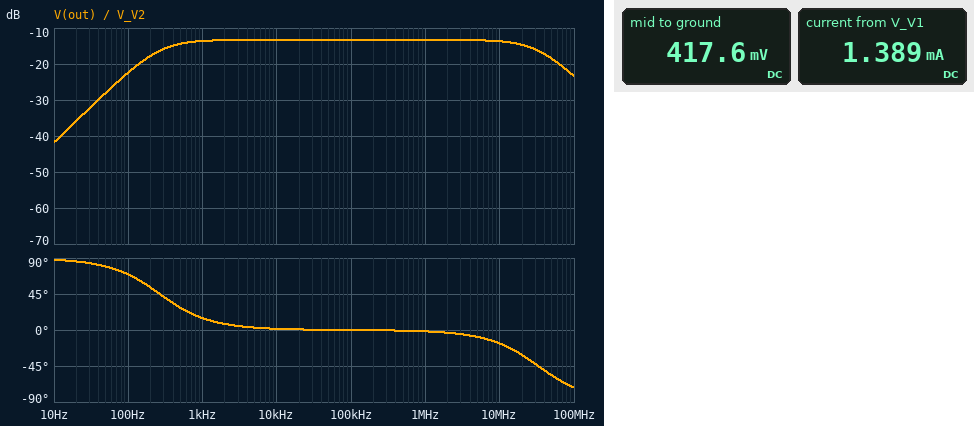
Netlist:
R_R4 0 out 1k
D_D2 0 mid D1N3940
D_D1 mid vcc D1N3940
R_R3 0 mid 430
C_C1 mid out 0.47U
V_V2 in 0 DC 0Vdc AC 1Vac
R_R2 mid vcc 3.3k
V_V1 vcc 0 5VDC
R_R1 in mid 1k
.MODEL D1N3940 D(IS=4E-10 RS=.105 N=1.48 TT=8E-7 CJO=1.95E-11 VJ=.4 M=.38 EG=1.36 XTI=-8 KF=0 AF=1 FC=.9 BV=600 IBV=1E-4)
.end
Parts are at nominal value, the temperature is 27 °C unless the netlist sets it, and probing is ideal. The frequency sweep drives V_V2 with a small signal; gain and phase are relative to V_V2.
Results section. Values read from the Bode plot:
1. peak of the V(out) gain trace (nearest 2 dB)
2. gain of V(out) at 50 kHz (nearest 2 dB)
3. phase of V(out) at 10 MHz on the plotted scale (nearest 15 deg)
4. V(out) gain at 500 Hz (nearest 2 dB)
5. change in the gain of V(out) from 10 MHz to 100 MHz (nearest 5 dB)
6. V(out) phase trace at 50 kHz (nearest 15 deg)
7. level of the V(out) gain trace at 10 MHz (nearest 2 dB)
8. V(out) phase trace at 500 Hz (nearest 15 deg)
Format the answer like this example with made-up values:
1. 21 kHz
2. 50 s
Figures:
1. -14 dB
2. -14 dB
3. -15 deg
4. -14 dB
5. -10 dB
6. 0 deg
7. -14 dB
8. 30 deg
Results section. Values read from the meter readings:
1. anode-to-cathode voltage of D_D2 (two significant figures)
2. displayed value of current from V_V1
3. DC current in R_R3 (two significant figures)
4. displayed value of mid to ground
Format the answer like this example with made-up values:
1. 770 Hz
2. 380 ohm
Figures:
1. -420 mV
2. 1.389 mA
3. 970 µA
4. 417.6 mV
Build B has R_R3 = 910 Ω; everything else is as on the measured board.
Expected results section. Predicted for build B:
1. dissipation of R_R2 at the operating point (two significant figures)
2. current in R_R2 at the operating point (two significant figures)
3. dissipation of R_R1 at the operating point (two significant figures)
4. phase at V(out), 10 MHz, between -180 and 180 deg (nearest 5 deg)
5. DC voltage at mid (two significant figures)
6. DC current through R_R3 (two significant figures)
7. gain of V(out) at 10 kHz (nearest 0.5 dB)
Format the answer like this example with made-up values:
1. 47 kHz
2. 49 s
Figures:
1. 5.8 mW
2. 1.3 mA
3. 400 µW
4. -20 deg
5. 630 mV
6. 690 µA
7. -10.5 dB
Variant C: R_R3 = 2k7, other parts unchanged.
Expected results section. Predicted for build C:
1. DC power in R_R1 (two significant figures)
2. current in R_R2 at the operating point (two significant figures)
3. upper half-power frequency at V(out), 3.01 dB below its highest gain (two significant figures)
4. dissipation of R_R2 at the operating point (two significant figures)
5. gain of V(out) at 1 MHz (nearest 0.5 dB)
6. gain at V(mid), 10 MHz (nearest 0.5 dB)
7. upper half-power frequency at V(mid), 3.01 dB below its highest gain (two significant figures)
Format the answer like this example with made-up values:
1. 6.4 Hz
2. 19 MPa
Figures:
1. 820 µW
2. 1.2 mA
3. 21 MHz
4. 5.1 mW
5. -8.5 dB
6. -9.5 dB
7. 460 Hz
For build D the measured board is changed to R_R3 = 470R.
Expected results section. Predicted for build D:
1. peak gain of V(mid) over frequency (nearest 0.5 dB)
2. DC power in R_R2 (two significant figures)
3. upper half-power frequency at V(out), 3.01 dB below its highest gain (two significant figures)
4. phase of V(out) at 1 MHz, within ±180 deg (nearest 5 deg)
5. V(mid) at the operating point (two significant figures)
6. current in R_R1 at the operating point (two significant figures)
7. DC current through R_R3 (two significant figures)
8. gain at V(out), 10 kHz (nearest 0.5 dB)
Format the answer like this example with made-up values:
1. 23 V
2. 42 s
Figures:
1. -10.5 dB
2. 6.3 mW
3. 32 MHz
4. 0 deg
5. 440 mV
6. 440 µA
7. 940 µA
8. -13.0 dB
